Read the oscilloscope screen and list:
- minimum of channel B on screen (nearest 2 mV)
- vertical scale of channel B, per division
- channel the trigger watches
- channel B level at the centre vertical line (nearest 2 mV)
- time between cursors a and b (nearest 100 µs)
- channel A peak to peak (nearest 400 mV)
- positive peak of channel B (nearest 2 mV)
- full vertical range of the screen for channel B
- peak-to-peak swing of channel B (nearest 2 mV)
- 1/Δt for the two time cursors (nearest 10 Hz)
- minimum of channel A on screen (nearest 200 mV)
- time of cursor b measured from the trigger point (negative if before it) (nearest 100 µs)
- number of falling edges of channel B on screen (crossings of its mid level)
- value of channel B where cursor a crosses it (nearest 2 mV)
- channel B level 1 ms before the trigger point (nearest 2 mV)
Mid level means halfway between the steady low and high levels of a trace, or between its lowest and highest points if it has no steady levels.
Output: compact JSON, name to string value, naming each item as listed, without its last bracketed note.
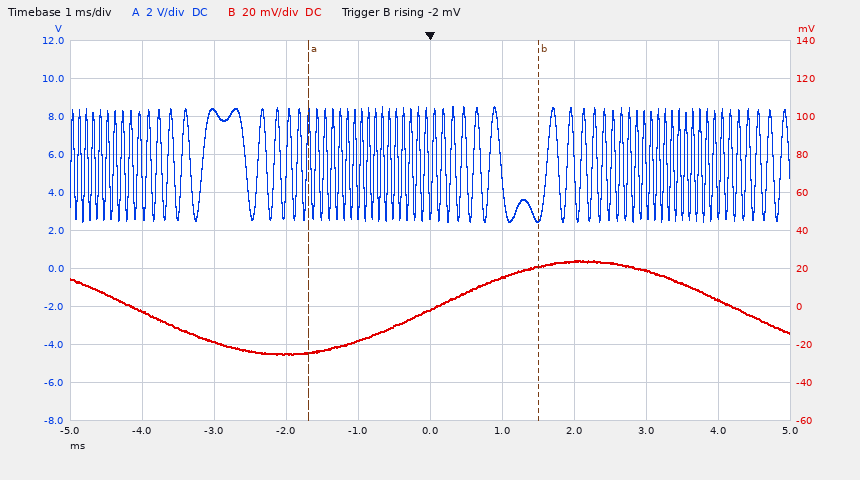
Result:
{"minimum of channel B on screen": "-26 mV", "vertical scale of channel B, per division": "20 mV", "channel the trigger watches": "channel B", "channel B level at the centre vertical line": "-2 mV", "time between cursors a and b": "3.2 ms", "channel A peak to peak": "6.0 V", "positive peak of channel B": "24 mV", "full vertical range of the screen for channel B": "200 mV", "peak-to-peak swing of channel B": "50 mV", "1/Δt for the two time cursors": "310 Hz", "minimum of channel A on screen": "2.4 V", "time of cursor b measured from the trigger point (negative if before it)": "+1.5 ms", "number of falling edges of channel B on screen": "2", "value of channel B where cursor a crosses it": "-24 mV", "channel B level 1 ms before the trigger point": "-18 mV"}
